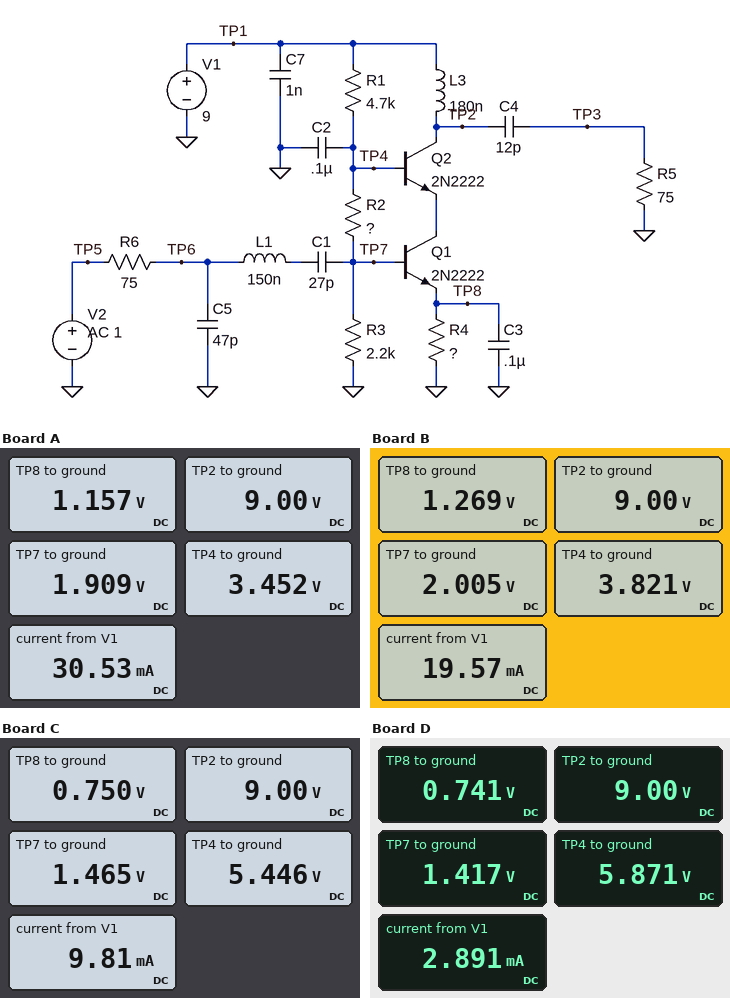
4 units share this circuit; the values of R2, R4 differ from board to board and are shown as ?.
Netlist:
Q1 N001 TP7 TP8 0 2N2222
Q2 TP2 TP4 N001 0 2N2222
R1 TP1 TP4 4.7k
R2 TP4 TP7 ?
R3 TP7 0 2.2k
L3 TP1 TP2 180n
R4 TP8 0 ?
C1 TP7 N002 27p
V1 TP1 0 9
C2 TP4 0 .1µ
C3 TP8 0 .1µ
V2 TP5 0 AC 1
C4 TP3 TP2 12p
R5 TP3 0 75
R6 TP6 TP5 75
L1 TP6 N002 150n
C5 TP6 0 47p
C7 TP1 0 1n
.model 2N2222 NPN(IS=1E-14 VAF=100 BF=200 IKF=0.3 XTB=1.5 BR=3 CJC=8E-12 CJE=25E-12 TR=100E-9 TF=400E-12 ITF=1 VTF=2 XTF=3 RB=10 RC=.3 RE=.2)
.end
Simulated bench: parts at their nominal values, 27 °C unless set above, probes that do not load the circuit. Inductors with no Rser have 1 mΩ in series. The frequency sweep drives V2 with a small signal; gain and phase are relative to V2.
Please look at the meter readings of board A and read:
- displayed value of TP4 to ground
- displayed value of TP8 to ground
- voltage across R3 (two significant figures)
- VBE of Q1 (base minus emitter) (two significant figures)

3.452 V
1.157 V
1.9 V
750 mV
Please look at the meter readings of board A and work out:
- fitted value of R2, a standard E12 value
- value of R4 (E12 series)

1.5 kΩ
39 Ω
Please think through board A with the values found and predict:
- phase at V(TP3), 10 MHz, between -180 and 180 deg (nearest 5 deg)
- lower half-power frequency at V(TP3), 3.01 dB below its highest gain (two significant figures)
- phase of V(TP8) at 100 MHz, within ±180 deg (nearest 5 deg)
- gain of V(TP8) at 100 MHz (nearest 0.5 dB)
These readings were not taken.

-10 deg
87 MHz
115 deg
-60.0 dB
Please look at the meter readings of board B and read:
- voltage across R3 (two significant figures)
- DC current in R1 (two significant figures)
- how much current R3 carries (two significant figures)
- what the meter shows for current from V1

2.0 V
1.1 mA
910 µA
19.57 mA
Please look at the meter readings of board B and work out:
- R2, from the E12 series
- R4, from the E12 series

1.8 kΩ
68 Ω
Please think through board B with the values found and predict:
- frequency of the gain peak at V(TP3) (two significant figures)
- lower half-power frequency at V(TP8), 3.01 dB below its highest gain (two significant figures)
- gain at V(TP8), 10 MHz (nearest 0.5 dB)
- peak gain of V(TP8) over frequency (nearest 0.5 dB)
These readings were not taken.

98 MHz
210 kHz
-42.5 dB
-29.0 dB
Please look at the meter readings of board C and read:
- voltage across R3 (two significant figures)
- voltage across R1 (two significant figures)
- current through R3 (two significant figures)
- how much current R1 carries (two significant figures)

1.5 V
3.6 V
670 µA
760 µA
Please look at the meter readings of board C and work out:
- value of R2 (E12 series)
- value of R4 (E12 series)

5.6 kΩ
82 Ω
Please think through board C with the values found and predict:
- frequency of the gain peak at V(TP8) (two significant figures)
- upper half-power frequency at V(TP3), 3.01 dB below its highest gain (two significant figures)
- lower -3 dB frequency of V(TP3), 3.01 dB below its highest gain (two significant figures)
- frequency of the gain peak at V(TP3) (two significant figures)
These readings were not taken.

540 kHz
110 MHz
88 MHz
99 MHz
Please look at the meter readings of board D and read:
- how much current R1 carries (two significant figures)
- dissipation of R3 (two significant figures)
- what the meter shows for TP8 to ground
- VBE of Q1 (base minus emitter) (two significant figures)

670 µA
910 µW
0.741 V
680 mV
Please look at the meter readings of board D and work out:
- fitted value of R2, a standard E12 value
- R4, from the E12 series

6.8 kΩ
330 Ω
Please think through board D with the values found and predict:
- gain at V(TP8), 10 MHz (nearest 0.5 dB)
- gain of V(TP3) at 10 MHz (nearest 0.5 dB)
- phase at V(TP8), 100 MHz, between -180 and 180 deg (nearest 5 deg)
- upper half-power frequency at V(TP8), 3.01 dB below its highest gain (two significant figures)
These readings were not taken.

-50.0 dB
-38.0 dB
170 deg
1.6 MHz
